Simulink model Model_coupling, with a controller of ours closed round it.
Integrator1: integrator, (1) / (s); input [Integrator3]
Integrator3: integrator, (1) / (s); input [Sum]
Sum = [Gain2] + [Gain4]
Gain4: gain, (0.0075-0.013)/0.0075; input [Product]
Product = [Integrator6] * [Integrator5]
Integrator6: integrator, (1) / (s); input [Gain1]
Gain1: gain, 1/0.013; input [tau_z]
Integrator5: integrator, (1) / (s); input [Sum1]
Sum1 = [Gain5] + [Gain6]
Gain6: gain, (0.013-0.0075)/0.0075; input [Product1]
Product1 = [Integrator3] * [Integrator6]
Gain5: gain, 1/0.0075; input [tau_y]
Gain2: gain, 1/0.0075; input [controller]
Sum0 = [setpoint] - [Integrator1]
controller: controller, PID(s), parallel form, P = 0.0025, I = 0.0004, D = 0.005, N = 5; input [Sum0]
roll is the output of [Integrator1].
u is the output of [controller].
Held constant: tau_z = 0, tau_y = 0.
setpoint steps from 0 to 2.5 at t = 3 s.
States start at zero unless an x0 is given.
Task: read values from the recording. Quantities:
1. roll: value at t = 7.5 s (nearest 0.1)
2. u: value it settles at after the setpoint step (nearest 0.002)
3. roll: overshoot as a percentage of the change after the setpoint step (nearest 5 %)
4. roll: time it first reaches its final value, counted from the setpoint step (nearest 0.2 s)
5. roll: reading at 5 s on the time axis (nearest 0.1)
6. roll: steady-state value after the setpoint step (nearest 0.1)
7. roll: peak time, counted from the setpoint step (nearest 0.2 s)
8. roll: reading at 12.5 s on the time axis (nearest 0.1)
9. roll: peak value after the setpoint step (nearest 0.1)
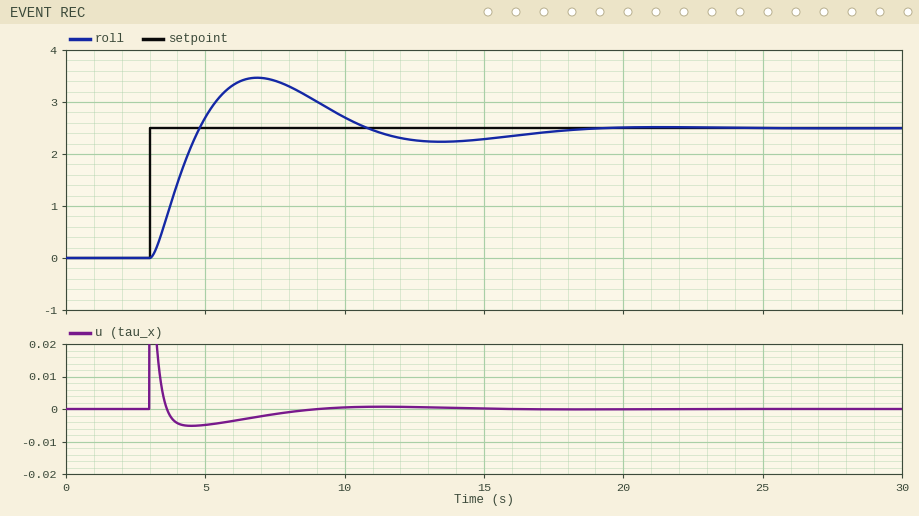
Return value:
3.4
0.000
40 %
1.8 s
2.7
2.5
3.8 s
2.3
3.5
